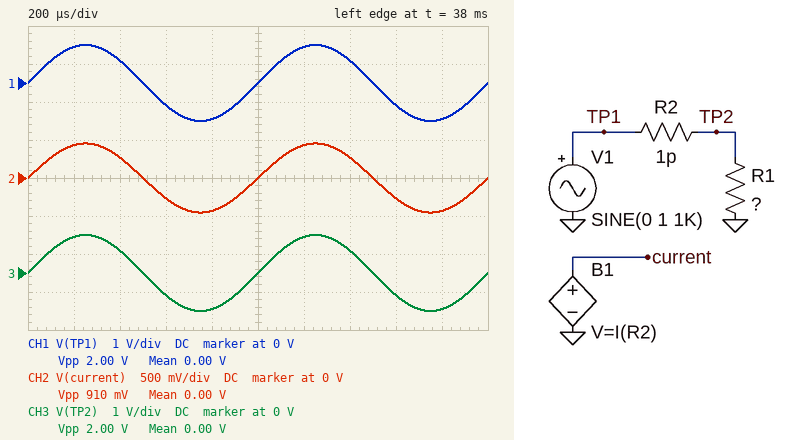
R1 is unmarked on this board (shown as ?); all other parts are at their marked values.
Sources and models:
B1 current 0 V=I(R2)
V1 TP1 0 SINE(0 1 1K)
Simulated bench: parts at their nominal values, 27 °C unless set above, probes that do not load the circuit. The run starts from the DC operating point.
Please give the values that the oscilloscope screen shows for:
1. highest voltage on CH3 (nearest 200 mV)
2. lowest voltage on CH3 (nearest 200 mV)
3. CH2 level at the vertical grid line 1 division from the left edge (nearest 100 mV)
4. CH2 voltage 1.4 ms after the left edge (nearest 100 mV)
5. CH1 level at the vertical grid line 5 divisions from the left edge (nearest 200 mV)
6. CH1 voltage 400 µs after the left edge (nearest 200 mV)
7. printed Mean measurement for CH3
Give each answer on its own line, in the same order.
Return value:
1.0 V
-1.0 V
400 mV
300 mV
0 V
600 mV
0.00 V
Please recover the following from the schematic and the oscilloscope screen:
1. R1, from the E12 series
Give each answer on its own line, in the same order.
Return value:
2.2 Ω
